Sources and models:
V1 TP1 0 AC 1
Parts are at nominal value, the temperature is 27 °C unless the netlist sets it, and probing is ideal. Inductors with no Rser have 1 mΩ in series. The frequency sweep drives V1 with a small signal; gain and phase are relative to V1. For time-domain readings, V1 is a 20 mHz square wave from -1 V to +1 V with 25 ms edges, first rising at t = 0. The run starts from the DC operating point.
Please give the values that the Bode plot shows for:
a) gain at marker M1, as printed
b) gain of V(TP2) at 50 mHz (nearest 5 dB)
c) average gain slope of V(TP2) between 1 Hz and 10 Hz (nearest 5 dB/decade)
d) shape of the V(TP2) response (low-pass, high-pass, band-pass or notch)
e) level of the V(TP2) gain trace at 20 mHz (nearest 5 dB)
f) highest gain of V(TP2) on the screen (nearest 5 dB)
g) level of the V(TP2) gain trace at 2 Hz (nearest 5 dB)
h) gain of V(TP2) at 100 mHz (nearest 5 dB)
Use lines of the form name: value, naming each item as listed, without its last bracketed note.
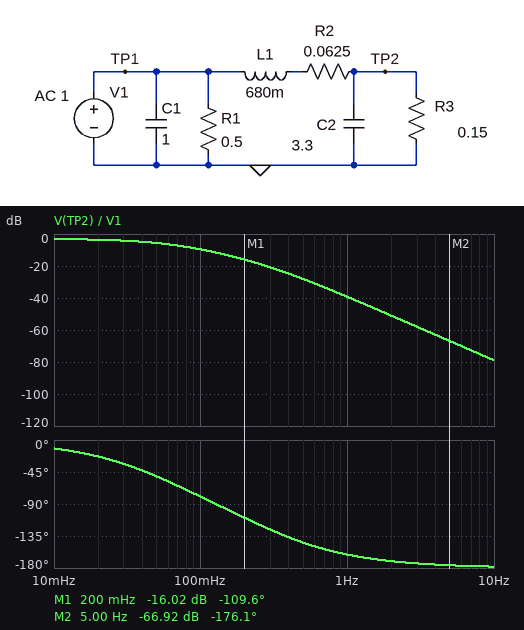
gain at marker M1, as printed: -16.02 dB
gain of V(TP2) at 50 mHz: -5 dB
average gain slope of V(TP2) between 1 Hz and 10 Hz: -40 dB/decade
shape of the V(TP2) response: low-pass
level of the V(TP2) gain trace at 20 mHz: -5 dB
highest gain of V(TP2) on the screen: -5 dB
level of the V(TP2) gain trace at 2 Hz: -50 dB
gain of V(TP2) at 100 mHz: -10 dB
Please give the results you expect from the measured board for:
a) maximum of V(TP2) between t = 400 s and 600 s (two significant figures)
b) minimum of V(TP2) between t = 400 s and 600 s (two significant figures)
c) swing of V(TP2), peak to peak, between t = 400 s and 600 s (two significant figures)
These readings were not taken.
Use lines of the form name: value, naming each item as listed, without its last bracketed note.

maximum of V(TP2) between t = 400 s and 600 s: 700 mV
minimum of V(TP2) between t = 400 s and 600 s: -700 mV
swing of V(TP2), peak to peak, between t = 400 s and 600 s: 1.4 V
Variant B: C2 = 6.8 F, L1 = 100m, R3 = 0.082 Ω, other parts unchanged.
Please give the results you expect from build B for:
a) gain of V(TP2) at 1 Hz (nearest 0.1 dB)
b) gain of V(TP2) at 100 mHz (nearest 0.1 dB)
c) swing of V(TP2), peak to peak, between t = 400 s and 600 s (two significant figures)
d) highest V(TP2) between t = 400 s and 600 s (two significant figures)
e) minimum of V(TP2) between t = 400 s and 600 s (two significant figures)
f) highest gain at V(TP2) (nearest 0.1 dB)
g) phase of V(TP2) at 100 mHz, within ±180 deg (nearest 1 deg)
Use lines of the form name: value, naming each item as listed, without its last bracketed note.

gain of V(TP2) at 1 Hz: -28.7 dB
gain of V(TP2) at 100 mHz: -5.2 dB
swing of V(TP2), peak to peak, between t = 400 s and 600 s: 1.2 V
highest V(TP2) between t = 400 s and 600 s: 600 mV
minimum of V(TP2) between t = 400 s and 600 s: -600 mV
highest gain at V(TP2): -5.0 dB
phase of V(TP2) at 100 mHz, within ±180 deg: -35 deg
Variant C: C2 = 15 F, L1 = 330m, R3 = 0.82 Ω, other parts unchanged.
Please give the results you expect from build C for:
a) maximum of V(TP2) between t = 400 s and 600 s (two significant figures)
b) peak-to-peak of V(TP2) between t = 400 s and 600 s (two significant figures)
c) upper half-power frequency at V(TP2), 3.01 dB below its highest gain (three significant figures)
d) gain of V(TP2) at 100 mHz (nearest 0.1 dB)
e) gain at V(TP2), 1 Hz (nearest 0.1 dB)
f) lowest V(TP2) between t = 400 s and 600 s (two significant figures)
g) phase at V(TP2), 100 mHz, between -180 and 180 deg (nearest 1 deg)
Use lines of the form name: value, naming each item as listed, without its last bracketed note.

maximum of V(TP2) between t = 400 s and 600 s: 1.6 V
peak-to-peak of V(TP2) between t = 400 s and 600 s: 3.3 V
upper half-power frequency at V(TP2), 3.01 dB below its highest gain: 87.5 mHz
gain of V(TP2) at 100 mHz: -1.7 dB
gain at V(TP2), 1 Hz: -45.8 dB
lowest V(TP2) between t = 400 s and 600 s: -1.6 V
phase at V(TP2), 100 mHz, between -180 and 180 deg: -136 deg
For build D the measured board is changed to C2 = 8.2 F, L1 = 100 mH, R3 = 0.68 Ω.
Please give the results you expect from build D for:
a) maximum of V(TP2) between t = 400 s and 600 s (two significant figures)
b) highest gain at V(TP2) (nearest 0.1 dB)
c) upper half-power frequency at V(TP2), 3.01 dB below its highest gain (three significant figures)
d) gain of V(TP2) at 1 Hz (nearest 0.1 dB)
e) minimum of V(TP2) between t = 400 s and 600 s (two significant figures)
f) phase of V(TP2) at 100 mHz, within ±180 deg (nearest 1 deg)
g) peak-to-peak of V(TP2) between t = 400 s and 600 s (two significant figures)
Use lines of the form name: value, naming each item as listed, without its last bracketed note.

maximum of V(TP2) between t = 400 s and 600 s: 1.5 V
highest gain at V(TP2): 2.8 dB
upper half-power frequency at V(TP2), 3.01 dB below its highest gain: 218 mHz
gain of V(TP2) at 1 Hz: -30.0 dB
minimum of V(TP2) between t = 400 s and 600 s: -1.5 V
phase of V(TP2) at 100 mHz, within ±180 deg: -29 deg
peak-to-peak of V(TP2) between t = 400 s and 600 s: 3.0 V
